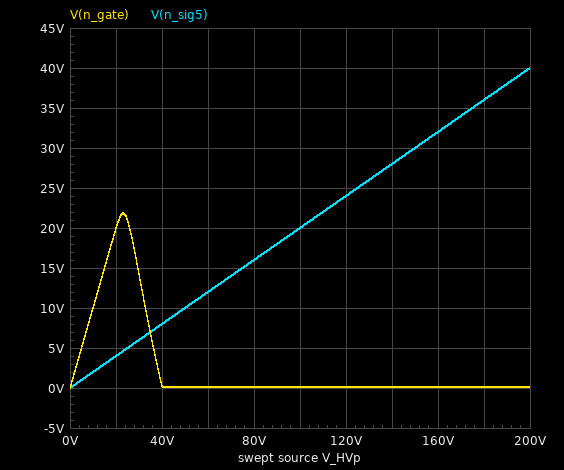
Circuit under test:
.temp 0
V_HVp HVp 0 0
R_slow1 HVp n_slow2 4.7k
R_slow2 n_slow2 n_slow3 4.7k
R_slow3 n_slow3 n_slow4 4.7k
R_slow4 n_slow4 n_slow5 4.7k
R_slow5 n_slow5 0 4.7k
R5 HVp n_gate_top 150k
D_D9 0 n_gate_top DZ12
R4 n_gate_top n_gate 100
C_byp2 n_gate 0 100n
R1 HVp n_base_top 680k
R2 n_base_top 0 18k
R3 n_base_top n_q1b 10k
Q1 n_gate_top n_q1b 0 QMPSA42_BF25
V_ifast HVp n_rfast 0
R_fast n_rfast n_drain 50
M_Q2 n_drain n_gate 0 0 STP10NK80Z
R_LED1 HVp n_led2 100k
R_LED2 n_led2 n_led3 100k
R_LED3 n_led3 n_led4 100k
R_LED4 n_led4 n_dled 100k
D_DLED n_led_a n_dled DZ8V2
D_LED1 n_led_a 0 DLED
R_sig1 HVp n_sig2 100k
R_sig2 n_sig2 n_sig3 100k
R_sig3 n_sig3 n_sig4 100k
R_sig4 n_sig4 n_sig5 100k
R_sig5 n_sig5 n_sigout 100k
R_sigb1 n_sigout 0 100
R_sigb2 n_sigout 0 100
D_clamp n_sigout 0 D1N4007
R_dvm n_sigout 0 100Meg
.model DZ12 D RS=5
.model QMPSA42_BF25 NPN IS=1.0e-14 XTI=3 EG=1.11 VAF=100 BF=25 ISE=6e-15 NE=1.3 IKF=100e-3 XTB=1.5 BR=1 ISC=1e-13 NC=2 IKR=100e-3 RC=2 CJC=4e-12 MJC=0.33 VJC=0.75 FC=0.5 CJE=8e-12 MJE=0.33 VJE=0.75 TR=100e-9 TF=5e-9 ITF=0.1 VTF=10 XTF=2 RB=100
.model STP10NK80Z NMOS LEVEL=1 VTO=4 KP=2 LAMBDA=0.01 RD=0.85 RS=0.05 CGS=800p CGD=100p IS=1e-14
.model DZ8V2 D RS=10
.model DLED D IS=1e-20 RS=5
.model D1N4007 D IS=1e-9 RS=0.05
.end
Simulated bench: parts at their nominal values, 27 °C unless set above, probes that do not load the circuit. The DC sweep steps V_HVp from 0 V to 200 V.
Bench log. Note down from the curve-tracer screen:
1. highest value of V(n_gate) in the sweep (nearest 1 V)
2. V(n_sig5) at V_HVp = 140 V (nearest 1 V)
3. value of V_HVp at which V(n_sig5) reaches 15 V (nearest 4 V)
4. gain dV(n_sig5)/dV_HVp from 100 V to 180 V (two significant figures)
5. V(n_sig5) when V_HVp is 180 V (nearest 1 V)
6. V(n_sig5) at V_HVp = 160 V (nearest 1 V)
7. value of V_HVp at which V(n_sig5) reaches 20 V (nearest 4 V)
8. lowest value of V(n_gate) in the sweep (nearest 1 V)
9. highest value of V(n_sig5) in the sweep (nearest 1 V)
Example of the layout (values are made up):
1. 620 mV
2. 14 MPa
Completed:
1. 22 V
2. 28 V
3. 76 V
4. 0.20 V/V
5. 36 V
6. 32 V
7. 100 V
8. 0 V
9. 40 V
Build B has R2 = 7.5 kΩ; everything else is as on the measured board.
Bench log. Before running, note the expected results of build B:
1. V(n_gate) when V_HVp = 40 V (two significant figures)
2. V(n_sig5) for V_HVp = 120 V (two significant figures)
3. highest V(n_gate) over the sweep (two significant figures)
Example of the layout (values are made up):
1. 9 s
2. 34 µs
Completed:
1. 40 V
2. 24 V
3. 53 V
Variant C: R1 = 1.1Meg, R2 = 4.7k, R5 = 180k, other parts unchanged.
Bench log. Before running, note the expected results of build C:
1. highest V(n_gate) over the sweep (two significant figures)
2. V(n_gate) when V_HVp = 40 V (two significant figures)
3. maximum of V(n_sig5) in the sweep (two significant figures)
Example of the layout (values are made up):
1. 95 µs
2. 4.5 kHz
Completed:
1. 140 V
2. 40 V
3. 40 V
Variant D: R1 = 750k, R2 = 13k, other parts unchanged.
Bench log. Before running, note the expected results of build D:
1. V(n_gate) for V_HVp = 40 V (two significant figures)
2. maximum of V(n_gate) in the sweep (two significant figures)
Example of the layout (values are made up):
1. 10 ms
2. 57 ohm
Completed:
1. 31 V
2. 34 V
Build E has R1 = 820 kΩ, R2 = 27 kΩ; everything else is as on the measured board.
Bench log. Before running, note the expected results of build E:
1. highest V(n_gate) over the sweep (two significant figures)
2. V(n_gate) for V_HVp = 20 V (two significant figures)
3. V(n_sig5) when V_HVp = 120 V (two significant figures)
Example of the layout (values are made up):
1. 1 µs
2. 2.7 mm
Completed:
1. 18 V
2. 17 V
3. 24 V
